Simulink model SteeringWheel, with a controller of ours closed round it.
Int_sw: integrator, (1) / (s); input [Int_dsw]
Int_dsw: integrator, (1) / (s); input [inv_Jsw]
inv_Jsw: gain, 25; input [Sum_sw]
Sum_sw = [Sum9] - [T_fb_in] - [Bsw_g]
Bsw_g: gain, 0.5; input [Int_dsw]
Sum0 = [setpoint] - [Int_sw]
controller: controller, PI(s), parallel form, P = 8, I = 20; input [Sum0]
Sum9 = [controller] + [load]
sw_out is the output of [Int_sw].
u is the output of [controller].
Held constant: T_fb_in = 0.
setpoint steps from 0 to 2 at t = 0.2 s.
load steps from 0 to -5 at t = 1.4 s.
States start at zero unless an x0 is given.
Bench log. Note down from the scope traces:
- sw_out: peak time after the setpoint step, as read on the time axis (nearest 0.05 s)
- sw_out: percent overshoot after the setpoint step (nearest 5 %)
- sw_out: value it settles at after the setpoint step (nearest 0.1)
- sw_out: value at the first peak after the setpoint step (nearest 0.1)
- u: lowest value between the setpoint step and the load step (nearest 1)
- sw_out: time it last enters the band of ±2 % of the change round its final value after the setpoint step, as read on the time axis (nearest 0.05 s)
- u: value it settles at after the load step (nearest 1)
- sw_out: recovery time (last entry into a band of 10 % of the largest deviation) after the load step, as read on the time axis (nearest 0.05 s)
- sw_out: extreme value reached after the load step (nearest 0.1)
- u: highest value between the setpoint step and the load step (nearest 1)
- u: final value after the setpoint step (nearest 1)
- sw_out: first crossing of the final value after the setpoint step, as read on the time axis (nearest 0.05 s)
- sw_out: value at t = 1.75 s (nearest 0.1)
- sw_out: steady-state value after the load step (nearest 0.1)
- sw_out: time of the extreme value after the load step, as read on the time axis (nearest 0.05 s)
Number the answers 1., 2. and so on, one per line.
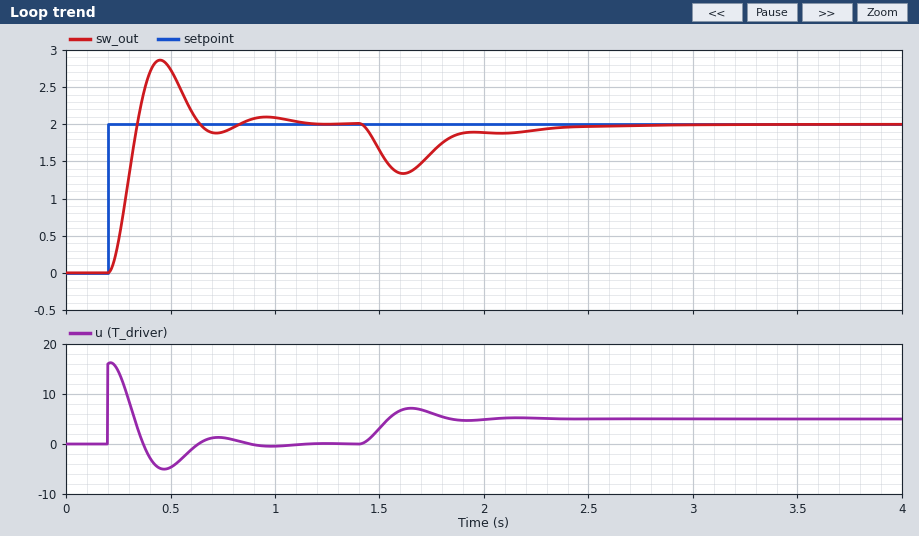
1. 0.45 s
2. 45 %
3. 2.0
4. 2.9
5. -5
6. 1.10 s
7. 5
8. 2.30 s
9. 1.3
10. 16
11. 0
12. 0.35 s
13. 1.6
14. 2.0
15. 1.60 s
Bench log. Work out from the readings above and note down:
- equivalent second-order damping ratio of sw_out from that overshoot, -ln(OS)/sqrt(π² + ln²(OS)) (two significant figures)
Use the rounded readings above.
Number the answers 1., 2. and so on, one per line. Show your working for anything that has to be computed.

1. ln(0.45) = -0.799; 0.799 / sqrt(9.870 + 0.638) = 0.25
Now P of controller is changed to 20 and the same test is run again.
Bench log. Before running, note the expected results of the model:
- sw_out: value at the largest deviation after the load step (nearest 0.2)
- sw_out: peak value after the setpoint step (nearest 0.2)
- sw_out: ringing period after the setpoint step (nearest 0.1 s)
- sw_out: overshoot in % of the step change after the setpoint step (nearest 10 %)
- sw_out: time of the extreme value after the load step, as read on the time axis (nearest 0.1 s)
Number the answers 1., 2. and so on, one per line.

1. 1.6
2. 3.0
3. 0.3 s
4. 50 %
5. 1.5 s
